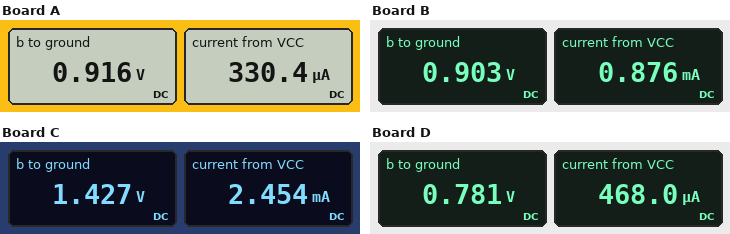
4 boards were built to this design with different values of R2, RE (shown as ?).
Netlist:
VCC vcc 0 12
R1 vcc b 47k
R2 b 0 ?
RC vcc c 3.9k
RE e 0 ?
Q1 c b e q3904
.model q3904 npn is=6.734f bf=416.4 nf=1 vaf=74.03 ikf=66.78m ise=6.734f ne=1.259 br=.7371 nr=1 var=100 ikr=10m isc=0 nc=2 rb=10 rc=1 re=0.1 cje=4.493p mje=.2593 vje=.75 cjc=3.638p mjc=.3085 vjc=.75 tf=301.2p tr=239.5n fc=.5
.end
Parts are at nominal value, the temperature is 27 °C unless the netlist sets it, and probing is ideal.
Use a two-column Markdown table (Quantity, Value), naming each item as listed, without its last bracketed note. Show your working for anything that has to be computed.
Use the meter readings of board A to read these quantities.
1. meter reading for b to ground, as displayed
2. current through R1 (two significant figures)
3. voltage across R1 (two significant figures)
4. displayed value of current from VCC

| Quantity | Value |
|---|---|
| meter reading for b to ground, as displayed | 0.916 V |
| current through R1 | (12 V - 916 mV) / 47 kΩ = 240 µA |
| voltage across R1 | 12 V - 916 mV = 11 V |
| displayed value of current from VCC | 330.4 µA |
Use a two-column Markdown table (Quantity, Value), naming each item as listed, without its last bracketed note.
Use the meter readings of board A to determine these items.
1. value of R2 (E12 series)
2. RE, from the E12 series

| Quantity | Value |
|---|---|
| value of R2 | 3.9 kΩ |
| RE, from the E12 series | 3.3 kΩ |
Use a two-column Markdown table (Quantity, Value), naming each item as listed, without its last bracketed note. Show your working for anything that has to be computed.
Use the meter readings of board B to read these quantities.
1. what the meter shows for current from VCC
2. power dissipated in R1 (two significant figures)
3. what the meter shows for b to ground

| Quantity | Value |
|---|---|
| what the meter shows for current from VCC | 0.876 mA |
| power dissipated in R1 | (12 V - 903 mV)^2 / 47 kΩ = 2.6 mW |
| what the meter shows for b to ground | 0.903 V |
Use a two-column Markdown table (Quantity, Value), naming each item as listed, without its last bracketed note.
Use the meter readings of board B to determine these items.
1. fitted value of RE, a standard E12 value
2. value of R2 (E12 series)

| Quantity | Value |
|---|---|
| fitted value of RE, a standard E12 value | 390 Ω |
| value of R2 | 3.9 kΩ |
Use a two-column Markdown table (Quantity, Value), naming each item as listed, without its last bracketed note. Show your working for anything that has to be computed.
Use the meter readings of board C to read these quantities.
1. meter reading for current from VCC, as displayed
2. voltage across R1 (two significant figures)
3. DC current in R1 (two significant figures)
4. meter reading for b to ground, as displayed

| Quantity | Value |
|---|---|
| meter reading for current from VCC, as displayed | 2.454 mA |
| voltage across R1 | 12 V - 1.427 V = 11 V |
| DC current in R1 | (12 V - 1.427 V) / 47 kΩ = 220 µA |
| meter reading for b to ground, as displayed | 1.427 V |
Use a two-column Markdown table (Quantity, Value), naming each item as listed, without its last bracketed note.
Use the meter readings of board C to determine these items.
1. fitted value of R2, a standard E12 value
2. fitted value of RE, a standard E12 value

| Quantity | Value |
|---|---|
| fitted value of R2, a standard E12 value | 6.8 kΩ |
| fitted value of RE, a standard E12 value | 330 Ω |
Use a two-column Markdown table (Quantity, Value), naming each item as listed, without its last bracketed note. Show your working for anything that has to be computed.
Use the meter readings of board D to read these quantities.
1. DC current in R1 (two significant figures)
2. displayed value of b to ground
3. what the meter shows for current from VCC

| Quantity | Value |
|---|---|
| DC current in R1 | (12 V - 781 mV) / 47 kΩ = 240 µA |
| displayed value of b to ground | 0.781 V |
| what the meter shows for current from VCC | 468.0 µA |
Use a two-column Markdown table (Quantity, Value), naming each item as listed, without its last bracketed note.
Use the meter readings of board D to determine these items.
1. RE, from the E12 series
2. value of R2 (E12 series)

| Quantity | Value |
|---|---|
| RE, from the E12 series | 680 Ω |
| value of R2 | 3.3 kΩ |
